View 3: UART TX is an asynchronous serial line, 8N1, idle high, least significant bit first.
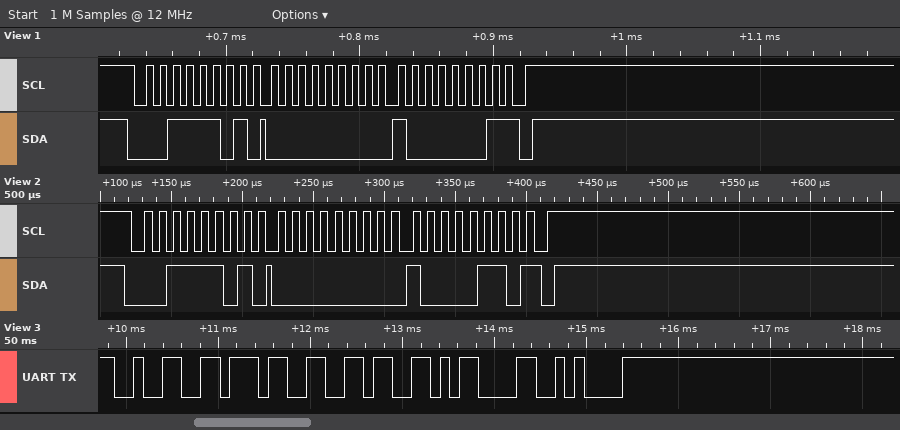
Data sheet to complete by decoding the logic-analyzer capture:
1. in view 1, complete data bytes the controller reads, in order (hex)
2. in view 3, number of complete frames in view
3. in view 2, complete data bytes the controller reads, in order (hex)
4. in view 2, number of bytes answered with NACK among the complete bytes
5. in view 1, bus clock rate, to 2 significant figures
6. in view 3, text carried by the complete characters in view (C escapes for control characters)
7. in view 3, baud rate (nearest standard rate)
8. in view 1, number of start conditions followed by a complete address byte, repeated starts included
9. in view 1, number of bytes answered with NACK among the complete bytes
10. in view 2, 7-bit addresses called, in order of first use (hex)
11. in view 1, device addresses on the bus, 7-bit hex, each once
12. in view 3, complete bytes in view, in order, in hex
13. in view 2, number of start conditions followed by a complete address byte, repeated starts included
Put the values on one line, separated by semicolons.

00 81; 5; 00 86; 1; 100 kHz; "276\r\n"; 9600 baud; 1; 1; 0x1E; 0x1E; 32 37 36 0D 0A; 1
